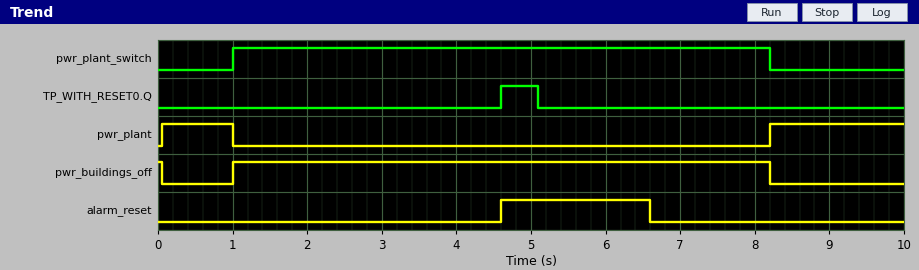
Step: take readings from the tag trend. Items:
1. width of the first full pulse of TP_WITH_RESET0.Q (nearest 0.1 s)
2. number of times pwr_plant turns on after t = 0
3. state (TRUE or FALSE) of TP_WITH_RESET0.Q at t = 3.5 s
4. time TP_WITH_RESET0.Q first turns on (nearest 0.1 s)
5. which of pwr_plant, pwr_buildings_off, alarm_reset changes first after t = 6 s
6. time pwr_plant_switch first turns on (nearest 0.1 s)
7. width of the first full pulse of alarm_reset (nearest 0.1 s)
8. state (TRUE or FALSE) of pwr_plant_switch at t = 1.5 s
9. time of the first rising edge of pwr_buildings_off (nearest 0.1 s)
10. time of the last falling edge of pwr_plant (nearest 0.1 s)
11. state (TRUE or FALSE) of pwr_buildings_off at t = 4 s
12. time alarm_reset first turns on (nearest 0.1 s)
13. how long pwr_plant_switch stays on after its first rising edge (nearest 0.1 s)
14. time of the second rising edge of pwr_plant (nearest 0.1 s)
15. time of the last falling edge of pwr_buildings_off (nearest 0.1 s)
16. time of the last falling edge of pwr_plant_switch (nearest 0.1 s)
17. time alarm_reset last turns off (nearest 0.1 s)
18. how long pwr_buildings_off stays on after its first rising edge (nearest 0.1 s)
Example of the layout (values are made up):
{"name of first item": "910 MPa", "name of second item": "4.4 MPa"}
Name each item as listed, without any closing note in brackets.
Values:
{"width of the first full pulse of TP_WITH_RESET0.Q": "0.5 s", "number of times pwr_plant turns on after t = 0": "2", "state (TRUE or FALSE) of TP_WITH_RESET0.Q at t = 3.5 s": "FALSE", "time TP_WITH_RESET0.Q first turns on": "4.6 s", "which of pwr_plant, pwr_buildings_off, alarm_reset changes first after t = 6 s": "alarm_reset", "time pwr_plant_switch first turns on": "1.0 s", "width of the first full pulse of alarm_reset": "2.0 s", "state (TRUE or FALSE) of pwr_plant_switch at t = 1.5 s": "TRUE", "time of the first rising edge of pwr_buildings_off": "1.0 s", "time of the last falling edge of pwr_plant": "1.0 s", "state (TRUE or FALSE) of pwr_buildings_off at t = 4 s": "TRUE", "time alarm_reset first turns on": "4.6 s", "how long pwr_plant_switch stays on after its first rising edge": "7.2 s", "time of the second rising edge of pwr_plant": "8.2 s", "time of the last falling edge of pwr_buildings_off": "8.2 s", "time of the last falling edge of pwr_plant_switch": "8.2 s", "time alarm_reset last turns off": "6.6 s", "how long pwr_buildings_off stays on after its first rising edge": "7.2 s"}
